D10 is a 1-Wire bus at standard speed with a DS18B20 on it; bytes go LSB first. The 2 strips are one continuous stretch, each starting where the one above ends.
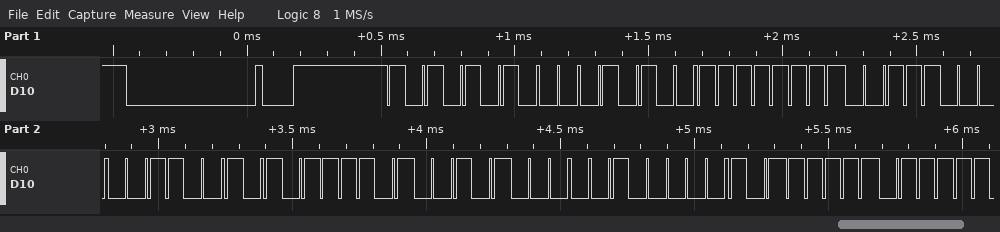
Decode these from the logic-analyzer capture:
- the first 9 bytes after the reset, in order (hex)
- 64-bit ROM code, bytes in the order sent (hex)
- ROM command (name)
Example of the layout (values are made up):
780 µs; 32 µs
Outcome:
55 28 FF 1C 4C BD 14 04 FD; 28 FF 1C 4C BD 14 04 FD; Match ROM
